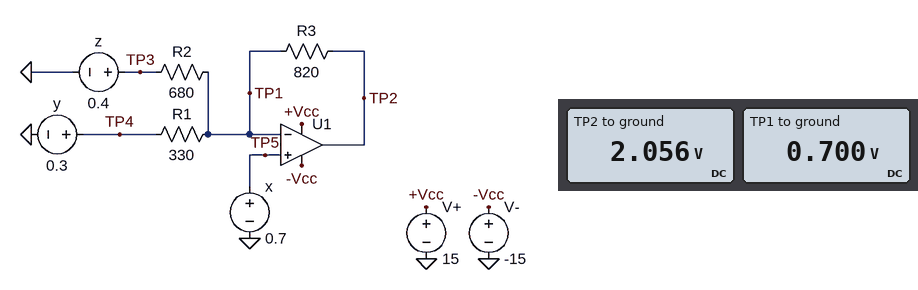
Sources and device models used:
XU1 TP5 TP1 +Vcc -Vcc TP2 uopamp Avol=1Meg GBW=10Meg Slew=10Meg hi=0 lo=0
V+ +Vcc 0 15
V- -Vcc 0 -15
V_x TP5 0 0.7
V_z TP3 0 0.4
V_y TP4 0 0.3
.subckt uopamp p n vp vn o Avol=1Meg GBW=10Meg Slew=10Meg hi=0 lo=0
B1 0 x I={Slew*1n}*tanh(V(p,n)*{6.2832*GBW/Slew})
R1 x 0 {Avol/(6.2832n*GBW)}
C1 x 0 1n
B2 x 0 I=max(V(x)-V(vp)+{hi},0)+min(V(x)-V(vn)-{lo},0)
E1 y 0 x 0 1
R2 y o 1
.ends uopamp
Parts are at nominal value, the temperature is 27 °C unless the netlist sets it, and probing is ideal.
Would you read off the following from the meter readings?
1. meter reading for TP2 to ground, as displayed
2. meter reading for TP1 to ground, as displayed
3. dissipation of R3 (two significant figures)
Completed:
2.056 V
0.700 V
2.2 mW
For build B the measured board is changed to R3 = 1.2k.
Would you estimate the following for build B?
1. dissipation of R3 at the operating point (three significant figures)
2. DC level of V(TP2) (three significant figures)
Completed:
3.28 mW
2.68 V
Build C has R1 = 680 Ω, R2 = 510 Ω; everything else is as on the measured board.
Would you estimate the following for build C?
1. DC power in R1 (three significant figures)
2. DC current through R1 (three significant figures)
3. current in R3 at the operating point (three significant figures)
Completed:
235 µW
588 µA
1.18 mA
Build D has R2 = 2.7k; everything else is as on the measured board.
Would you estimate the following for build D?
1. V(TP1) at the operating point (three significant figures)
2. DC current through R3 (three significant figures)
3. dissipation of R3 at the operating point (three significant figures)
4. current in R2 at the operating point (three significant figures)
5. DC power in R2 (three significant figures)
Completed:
700 mV
1.32 mA
1.44 mW
111 µA
33.3 µW
